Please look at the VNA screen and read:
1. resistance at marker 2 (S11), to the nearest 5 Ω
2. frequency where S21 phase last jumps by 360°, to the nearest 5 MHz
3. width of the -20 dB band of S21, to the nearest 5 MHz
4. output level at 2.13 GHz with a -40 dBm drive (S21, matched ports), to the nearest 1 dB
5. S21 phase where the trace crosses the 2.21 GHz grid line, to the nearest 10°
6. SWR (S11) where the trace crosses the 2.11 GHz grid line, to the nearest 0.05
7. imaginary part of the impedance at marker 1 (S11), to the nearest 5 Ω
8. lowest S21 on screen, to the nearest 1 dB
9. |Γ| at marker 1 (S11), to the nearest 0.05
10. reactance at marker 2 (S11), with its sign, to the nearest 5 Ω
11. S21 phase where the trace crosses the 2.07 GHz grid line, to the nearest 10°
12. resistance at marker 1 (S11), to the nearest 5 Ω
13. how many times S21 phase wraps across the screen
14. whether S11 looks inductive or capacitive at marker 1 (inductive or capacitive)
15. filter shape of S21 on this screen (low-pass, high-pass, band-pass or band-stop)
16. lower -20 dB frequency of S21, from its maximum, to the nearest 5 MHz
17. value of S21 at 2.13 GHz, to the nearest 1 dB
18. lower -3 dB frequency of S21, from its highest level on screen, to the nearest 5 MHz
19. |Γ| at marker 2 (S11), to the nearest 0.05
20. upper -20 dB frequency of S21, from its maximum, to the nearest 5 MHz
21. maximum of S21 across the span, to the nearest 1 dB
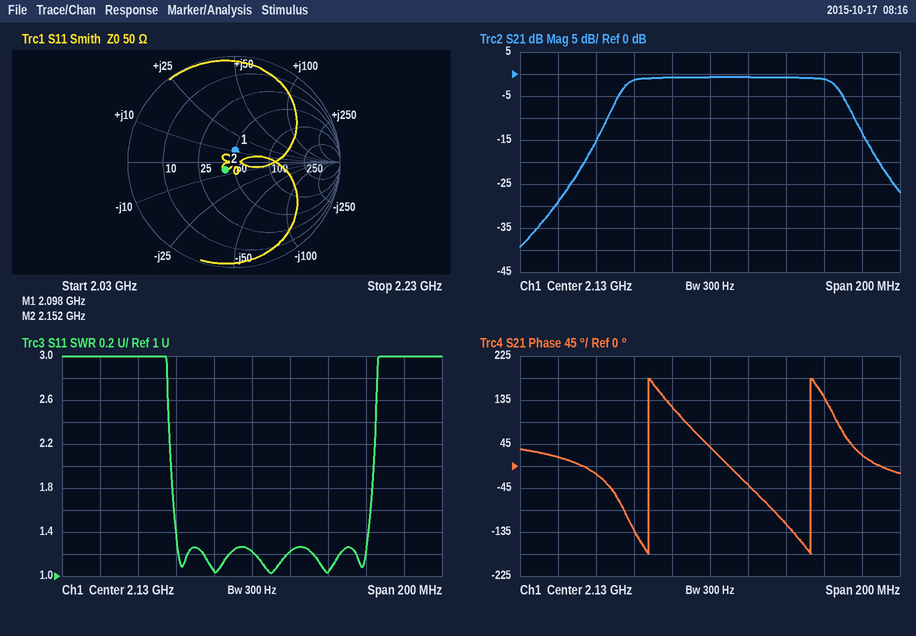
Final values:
40 Ω
2.185 GHz
155 MHz
-41 dBm
20°
1.05
+10 Ω
-39 dB
0.10
-5 Ω
-20°
50 Ω
2
inductive
band-pass
2.065 GHz
-1 dB
2.085 GHz
0.10
2.220 GHz
-1 dB
